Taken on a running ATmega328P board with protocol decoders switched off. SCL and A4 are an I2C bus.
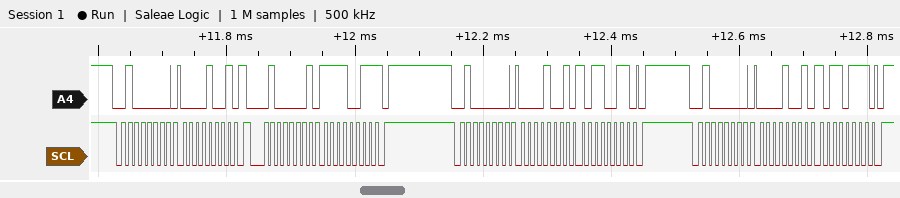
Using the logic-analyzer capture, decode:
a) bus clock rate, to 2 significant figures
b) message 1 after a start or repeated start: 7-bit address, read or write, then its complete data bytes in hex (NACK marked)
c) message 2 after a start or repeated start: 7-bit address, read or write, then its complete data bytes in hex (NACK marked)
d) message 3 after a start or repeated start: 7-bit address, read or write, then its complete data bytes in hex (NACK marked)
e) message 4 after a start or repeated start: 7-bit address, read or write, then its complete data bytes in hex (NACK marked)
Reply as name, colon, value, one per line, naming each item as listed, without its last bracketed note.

bus clock rate, to 2 significant figures: 100 kHz
message 1 after a start or repeated start: 7-bit address, read or write, then its complete data bytes in hex: 0x20 write: 09
message 2 after a start or repeated start: 7-bit address, read or write, then its complete data bytes in hex: 0x20 read: F3 NACK
message 3 after a start or repeated start: 7-bit address, read or write, then its complete data bytes in hex: 0x20 write: 09 B3
message 4 after a start or repeated start: 7-bit address, read or write, then its complete data bytes in hex: 0x20 write: 09 B7
